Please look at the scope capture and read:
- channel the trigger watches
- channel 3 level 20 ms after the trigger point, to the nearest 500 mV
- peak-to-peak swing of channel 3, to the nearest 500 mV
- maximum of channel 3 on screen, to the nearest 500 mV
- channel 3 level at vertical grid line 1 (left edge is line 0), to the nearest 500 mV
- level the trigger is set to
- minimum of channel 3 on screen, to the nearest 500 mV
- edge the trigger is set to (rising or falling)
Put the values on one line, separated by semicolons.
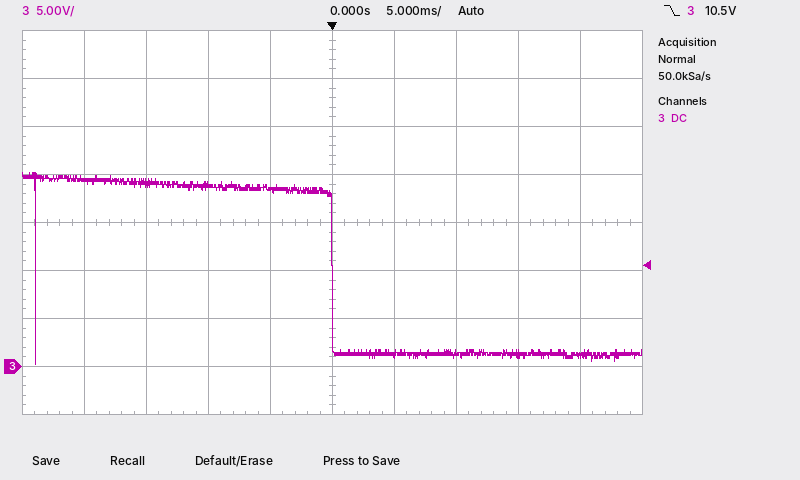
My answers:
channel 3; 1.0 V; 20.0 V; 20.0 V; 19.5 V; 10.5 V; 0.0 V; falling
